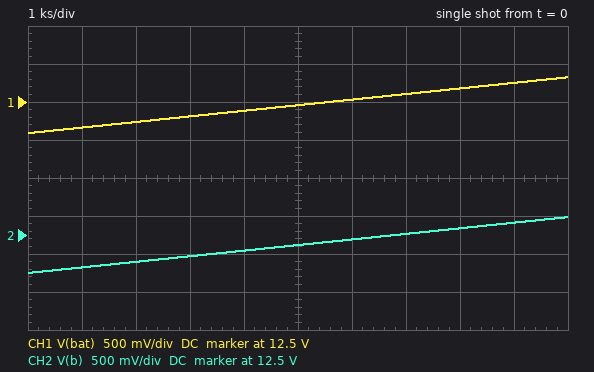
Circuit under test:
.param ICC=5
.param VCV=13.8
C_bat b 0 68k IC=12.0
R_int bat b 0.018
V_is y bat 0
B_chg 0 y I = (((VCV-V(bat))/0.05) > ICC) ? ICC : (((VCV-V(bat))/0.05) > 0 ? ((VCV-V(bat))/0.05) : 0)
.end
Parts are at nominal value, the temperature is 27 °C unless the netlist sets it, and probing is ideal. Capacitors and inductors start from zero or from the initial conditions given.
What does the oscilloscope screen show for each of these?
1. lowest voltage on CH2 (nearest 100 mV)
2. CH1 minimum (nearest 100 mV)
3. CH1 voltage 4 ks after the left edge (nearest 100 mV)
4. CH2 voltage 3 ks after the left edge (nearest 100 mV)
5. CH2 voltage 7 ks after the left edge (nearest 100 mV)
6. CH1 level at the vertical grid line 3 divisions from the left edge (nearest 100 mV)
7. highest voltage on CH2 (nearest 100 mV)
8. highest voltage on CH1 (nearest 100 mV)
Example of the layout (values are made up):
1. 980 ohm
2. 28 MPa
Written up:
1. 12.0 V
2. 12.1 V
3. 12.4 V
4. 12.2 V
5. 12.5 V
6. 12.3 V
7. 12.7 V
8. 12.8 V
